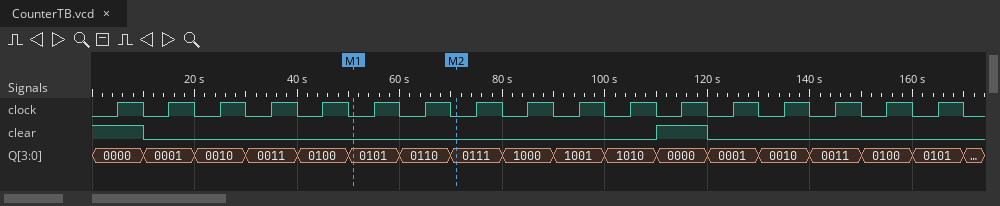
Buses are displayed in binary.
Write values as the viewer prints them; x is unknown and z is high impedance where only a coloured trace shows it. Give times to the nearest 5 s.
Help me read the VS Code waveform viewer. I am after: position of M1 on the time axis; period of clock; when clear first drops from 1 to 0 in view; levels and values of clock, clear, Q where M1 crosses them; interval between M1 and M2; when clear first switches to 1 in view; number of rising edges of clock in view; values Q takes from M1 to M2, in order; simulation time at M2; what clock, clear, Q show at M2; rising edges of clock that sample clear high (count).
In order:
50 s
10 s
10 s
clock=0, clear=0, Q=0101
20 s
110 s
17
0101, 0110, 0111
70 s
clock=0, clear=0, Q=0111
2
